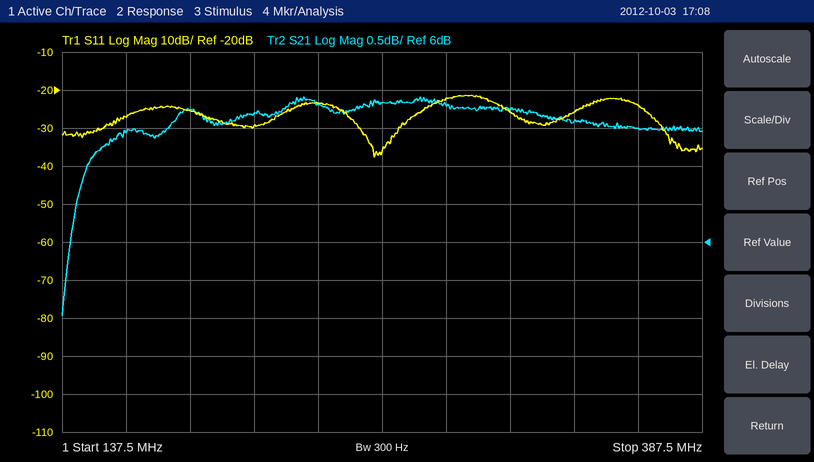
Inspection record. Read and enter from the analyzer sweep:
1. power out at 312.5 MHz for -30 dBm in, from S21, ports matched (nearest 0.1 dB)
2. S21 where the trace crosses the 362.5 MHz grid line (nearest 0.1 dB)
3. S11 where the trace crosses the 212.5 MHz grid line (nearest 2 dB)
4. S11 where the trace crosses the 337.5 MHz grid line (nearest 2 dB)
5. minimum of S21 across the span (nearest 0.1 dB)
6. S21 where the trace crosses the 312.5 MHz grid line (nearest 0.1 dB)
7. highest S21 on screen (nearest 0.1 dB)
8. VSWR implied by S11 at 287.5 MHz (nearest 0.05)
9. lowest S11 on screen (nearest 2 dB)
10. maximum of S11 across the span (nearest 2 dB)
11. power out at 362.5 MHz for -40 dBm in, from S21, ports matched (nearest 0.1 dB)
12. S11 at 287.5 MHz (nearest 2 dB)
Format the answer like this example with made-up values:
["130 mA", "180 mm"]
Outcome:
["-22.3 dBm", "7.5 dB", "-30 dB", "-26 dB", "5.0 dB", "7.7 dB", "7.9 dB", "1.15", "-38 dB", "-22 dB", "-32.5 dBm", "-22 dB"]
